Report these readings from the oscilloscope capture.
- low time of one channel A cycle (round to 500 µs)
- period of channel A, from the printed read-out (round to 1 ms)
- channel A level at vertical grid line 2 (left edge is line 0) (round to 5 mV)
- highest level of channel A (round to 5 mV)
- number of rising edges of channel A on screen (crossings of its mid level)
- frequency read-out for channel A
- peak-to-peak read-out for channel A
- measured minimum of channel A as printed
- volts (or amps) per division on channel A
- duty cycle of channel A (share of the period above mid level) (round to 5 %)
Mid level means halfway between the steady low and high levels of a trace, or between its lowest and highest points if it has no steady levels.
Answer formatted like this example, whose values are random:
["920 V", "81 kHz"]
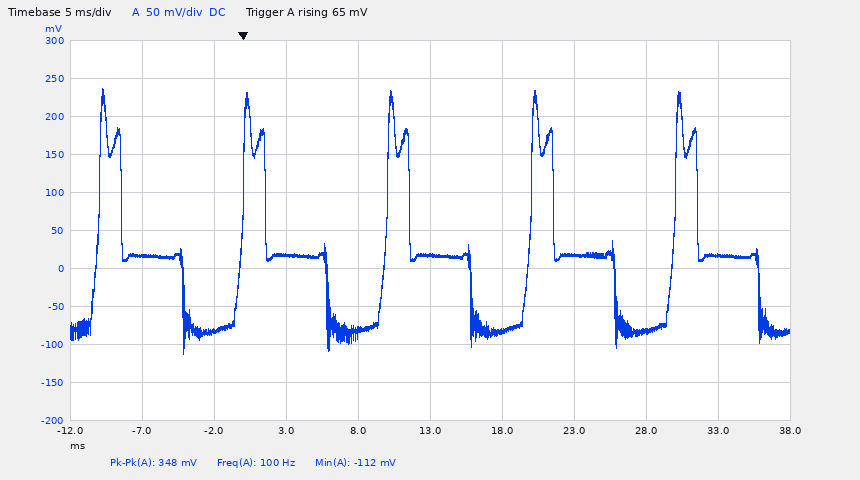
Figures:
["8.5 ms", "10 ms", "-85 mV", "235 mV", "5", "100 Hz", "348 mV", "-112 mV", "50 mV", "15 %"]
